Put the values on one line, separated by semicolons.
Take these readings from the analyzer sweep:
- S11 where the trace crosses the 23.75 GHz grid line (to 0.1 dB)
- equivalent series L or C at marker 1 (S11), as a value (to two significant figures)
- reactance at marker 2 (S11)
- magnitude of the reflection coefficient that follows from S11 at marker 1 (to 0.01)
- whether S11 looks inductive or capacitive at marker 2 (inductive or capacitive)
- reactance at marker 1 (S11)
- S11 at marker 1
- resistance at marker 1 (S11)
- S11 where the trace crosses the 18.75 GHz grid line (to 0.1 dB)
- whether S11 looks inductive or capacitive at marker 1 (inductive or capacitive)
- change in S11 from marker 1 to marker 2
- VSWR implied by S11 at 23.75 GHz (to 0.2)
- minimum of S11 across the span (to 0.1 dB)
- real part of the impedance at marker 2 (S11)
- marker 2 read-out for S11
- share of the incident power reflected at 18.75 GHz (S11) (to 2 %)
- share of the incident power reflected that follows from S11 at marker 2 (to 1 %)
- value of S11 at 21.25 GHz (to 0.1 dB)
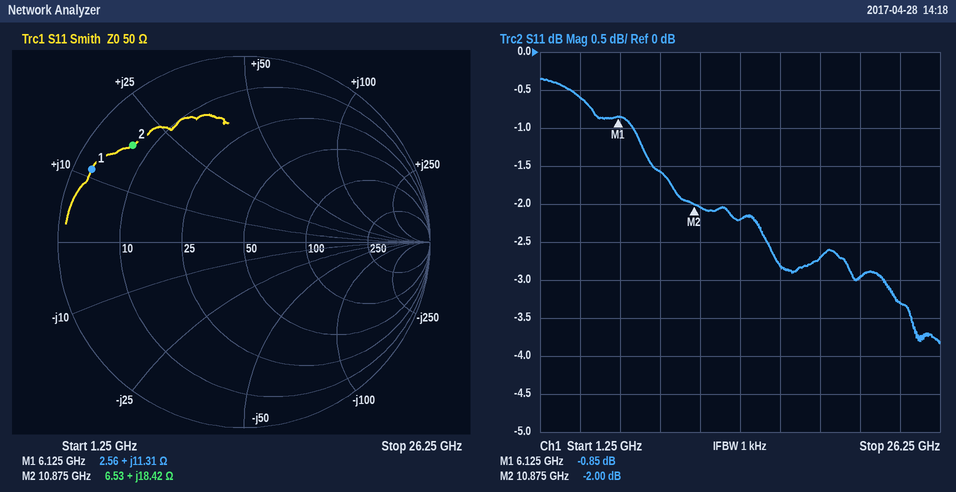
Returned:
-3.3 dB; 290 pH; +18.42 Ω; 0.91; inductive; +11.31 Ω; -0.85 dB; 2.56 Ω; -2.7 dB; inductive; -1.15 dB; 5.4; -3.8 dB; 6.53 Ω; -2.00 dB; 54 %; 63 %; -3.0 dB
